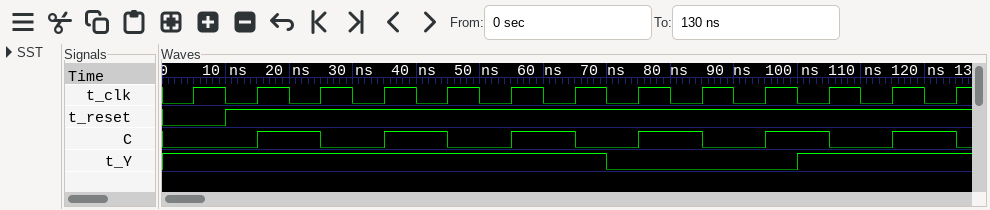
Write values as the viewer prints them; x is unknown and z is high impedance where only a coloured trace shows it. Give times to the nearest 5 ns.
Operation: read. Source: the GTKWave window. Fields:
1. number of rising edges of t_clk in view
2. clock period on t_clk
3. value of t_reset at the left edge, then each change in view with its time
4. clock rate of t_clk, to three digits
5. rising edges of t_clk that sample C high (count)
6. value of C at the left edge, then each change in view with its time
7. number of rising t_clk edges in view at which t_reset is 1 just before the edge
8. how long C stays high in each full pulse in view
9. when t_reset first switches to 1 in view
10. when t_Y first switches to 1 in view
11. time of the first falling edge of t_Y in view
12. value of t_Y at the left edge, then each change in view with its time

13
10 ns
0, 1 at 10 ns
100 MHz
6
0, 1 at 15 ns, 0 at 25 ns, 1 at 35 ns, 0 at 45 ns, 1 at 55 ns, 0 at 65 ns, 1 at 75 ns, 0 at 85 ns, 1 at 95 ns, 0 at 105 ns, 1 at 115 ns, 0 at 125 ns
12
10 ns, 10 ns, 10 ns, 10 ns, 10 ns, 10 ns
10 ns
100 ns
70 ns
1, 0 at 70 ns, 1 at 100 ns
